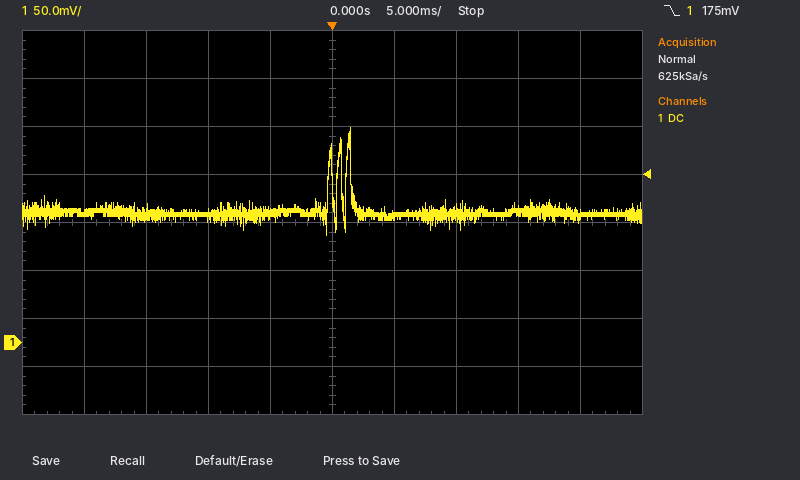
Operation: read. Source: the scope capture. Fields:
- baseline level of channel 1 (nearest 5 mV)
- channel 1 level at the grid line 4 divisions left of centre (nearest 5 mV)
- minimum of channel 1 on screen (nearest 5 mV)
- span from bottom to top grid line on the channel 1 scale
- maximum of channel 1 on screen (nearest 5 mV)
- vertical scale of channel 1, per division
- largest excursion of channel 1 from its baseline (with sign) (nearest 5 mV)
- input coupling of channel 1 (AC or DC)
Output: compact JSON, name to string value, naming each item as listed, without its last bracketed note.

{"baseline level of channel 1": "135 mV", "channel 1 level at the grid line 4 divisions left of centre": "135 mV", "minimum of channel 1 on screen": "110 mV", "span from bottom to top grid line on the channel 1 scale": "400 mV", "maximum of channel 1 on screen": "225 mV", "vertical scale of channel 1, per division": "50 mV", "largest excursion of channel 1 from its baseline (with sign)": "+90 mV", "input coupling of channel 1": "DC"}
